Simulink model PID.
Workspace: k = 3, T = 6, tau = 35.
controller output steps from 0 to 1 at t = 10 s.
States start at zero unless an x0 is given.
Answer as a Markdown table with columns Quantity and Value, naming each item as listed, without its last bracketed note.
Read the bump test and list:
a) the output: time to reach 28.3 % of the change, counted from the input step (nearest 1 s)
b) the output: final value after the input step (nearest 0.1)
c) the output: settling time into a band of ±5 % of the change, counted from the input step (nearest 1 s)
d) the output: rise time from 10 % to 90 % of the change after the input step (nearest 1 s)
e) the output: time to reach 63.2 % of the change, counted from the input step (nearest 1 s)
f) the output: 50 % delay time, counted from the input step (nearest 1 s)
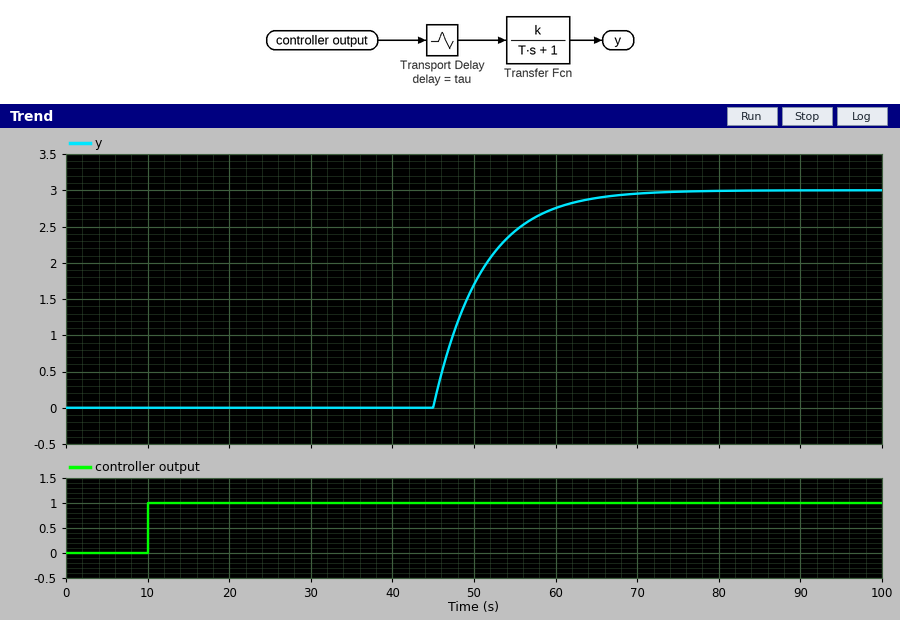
| Quantity | Value |
|---|---|
| the output: time to reach 28.3 % of the change, counted from the input step | 37 s |
| the output: final value after the input step | 3.0 |
| the output: settling time into a band of ±5 % of the change, counted from the input step | 53 s |
| the output: rise time from 10 % to 90 % of the change after the input step | 13 s |
| the output: time to reach 63.2 % of the change, counted from the input step | 41 s |
| the output: 50 % delay time, counted from the input step | 39 s |
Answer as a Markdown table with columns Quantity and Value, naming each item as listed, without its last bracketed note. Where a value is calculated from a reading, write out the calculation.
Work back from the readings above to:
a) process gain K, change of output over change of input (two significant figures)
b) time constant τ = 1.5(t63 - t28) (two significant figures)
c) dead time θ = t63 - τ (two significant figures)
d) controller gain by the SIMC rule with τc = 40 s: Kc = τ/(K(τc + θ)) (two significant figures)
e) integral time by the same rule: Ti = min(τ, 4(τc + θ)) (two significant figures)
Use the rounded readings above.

| Quantity | Value |
|---|---|
| process gain K, change of output over change of input | (3 - 0) / 1 = 3.0 |
| time constant τ = 1.5(t63 - t28) | 1.5 × (41 - 37) = 6.0 s |
| dead time θ = t63 - τ | 41 - 6 = 35 s |
| controller gain by the SIMC rule with τc = 40 s: Kc = τ/(K(τc + θ)) | 6 / (3 × (40 + 35)) = 0.027 |
| integral time by the same rule: Ti = min(τ, 4(τc + θ)) | min(6, 4 × (40 + 35)) = 6.0 s |
